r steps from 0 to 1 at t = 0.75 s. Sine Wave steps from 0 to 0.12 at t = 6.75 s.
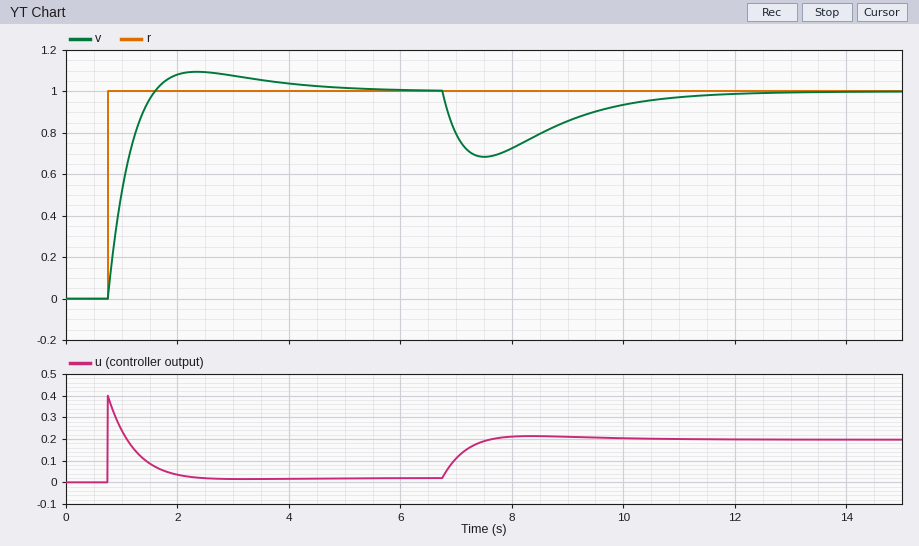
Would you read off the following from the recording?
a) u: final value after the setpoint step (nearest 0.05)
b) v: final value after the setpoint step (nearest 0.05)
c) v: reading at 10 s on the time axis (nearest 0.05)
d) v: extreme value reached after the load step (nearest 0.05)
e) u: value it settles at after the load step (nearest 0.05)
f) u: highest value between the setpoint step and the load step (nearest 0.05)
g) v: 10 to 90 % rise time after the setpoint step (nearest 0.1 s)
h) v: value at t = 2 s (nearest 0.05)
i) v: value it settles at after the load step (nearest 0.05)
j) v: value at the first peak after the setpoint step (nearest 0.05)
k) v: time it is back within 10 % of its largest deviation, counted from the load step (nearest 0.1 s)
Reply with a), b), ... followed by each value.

a) 0.00
b) 1.00
c) 0.95
d) 0.70
e) 0.20
f) 0.40
g) 0.6 s
h) 1.10
i) 1.00
j) 1.10
k) 4.1 s
